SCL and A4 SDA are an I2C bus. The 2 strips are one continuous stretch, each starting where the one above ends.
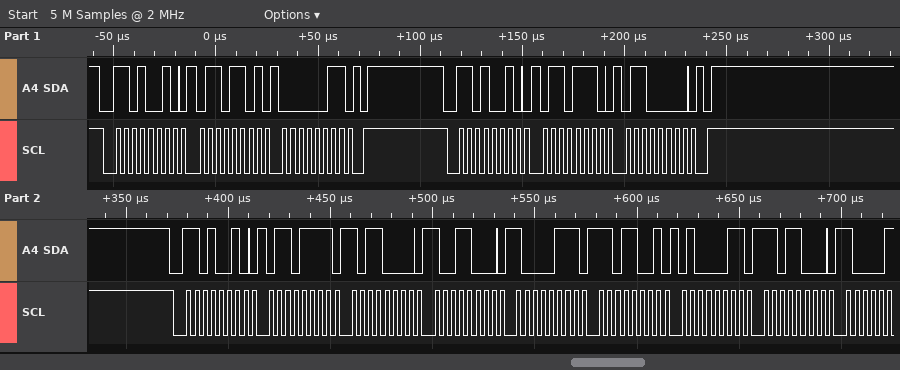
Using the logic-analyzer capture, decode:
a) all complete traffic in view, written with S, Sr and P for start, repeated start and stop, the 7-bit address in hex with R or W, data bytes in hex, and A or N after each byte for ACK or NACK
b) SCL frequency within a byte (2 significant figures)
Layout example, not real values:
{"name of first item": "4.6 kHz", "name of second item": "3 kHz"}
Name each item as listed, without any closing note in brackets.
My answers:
{"all complete traffic in view, written with S, Sr and P for start, repeated start and stop, the 7-bit address in hex with R or W, data bytes in hex, and A or N after each byte for ACK or NACK": "S 69W A 6D A 03 A P S 69W A 6E A 60 A P S 69W A 6F A B0 A 98 A 87 A D9 A 43 A D8 A", "SCL frequency within a byte": "250 kHz"}
